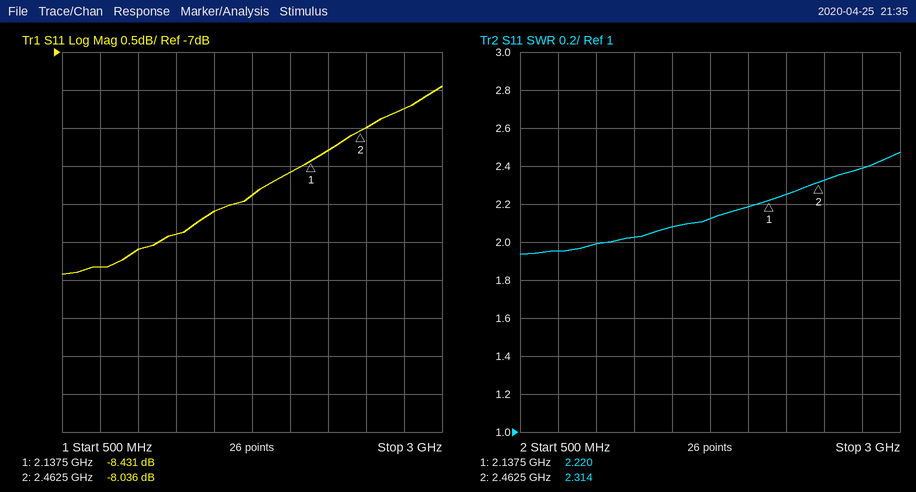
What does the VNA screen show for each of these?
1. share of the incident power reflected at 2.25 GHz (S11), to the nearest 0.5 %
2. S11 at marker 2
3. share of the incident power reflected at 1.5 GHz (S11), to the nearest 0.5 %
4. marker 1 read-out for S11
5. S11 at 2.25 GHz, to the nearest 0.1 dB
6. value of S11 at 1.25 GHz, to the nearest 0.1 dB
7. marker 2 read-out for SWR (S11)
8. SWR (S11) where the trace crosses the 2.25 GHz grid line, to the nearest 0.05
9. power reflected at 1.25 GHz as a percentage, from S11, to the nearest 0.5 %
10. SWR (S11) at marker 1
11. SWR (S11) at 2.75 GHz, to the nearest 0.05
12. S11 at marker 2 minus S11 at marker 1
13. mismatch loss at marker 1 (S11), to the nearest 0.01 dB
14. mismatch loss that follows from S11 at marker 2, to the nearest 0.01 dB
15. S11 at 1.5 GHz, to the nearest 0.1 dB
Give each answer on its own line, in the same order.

15.0 %
-8.036 dB
12.5 %
-8.431 dB
-8.3 dB
-9.4 dB
2.314
2.25
11.5 %
2.220
2.40
0.395 dB
0.67 dB
0.74 dB
-9.1 dB
